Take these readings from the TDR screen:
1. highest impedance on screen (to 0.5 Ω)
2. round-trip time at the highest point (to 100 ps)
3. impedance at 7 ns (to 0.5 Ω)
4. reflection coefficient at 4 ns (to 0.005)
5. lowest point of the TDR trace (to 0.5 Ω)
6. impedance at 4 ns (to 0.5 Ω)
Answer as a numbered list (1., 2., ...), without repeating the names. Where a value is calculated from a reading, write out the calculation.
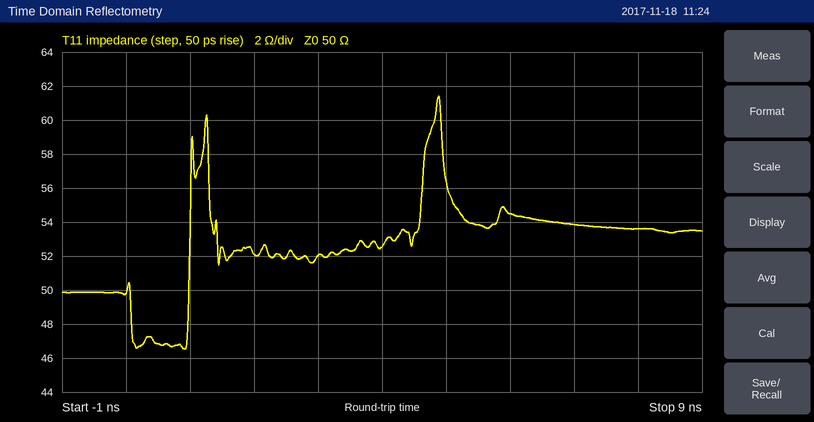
1. 61.5 Ω
2. 4.9 ns
3. 54.0 Ω
4. (52.5 − 50)/(52.5 + 50) ≈ +0.0244, so +0.025 to the nearest 0.005
5. 46.5 Ω
6. 52.5 Ω
